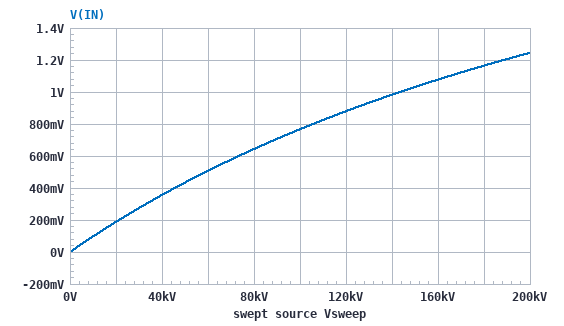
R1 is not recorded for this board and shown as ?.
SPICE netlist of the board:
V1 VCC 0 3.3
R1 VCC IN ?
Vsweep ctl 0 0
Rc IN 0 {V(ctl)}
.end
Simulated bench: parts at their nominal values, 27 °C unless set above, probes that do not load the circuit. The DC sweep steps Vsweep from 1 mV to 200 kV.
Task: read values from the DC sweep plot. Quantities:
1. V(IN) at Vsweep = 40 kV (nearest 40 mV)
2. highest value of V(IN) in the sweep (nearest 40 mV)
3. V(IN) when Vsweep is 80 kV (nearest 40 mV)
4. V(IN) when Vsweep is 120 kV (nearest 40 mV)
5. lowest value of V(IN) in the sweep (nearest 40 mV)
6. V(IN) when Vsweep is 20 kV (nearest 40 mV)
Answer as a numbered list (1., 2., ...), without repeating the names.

1. 360 mV
2. 1.24 V
3. 640 mV
4. 880 mV
5. 0 V
6. 200 mV
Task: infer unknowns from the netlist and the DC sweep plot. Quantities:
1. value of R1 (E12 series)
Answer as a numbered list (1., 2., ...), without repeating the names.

1. 330 kΩ
